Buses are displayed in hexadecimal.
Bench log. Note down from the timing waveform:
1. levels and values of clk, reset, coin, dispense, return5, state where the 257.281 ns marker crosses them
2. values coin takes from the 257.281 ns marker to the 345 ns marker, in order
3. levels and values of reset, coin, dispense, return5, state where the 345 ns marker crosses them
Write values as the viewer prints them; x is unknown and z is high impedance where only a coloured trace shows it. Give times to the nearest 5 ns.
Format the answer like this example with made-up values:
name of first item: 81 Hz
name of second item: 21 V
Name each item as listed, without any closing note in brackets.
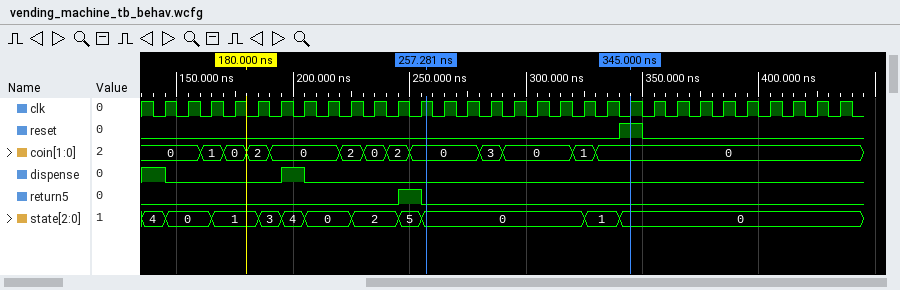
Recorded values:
levels and values of clk, reset, coin, dispense, return5, state where the 257.281 ns marker crosses them: clk=1, reset=0, coin=0, dispense=0, return5=0, state=0
values coin takes from the 257.281 ns marker to the 345 ns marker, in order: 0, 3, 0, 1, 0
levels and values of reset, coin, dispense, return5, state where the 345 ns marker crosses them: reset=1, coin=0, dispense=0, return5=0, state=0
